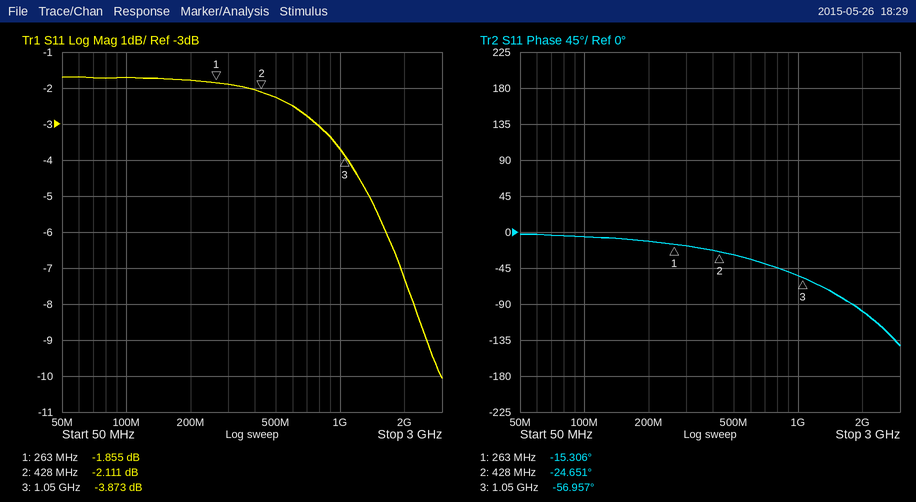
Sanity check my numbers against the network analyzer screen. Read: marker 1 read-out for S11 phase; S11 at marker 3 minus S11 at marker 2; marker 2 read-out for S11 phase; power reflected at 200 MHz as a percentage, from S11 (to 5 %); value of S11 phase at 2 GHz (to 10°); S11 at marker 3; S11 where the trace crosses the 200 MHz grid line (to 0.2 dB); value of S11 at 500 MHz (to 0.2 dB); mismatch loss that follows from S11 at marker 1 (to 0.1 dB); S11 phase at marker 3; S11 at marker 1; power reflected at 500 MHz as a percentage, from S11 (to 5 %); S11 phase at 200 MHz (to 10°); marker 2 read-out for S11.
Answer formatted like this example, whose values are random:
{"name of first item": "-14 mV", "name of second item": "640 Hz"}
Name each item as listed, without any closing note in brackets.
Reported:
{"marker 1 read-out for S11 phase": "-15.306°", "S11 at marker 3 minus S11 at marker 2": "-1.762 dB", "marker 2 read-out for S11 phase": "-24.651°", "power reflected at 200 MHz as a percentage, from S11": "65 %", "value of S11 phase at 2 GHz": "-100°", "S11 at marker 3": "-3.873 dB", "S11 where the trace crosses the 200 MHz grid line": "-1.8 dB", "value of S11 at 500 MHz": "-2.2 dB", "mismatch loss that follows from S11 at marker 1": "4.6 dB", "S11 phase at marker 3": "-56.957°", "S11 at marker 1": "-1.855 dB", "power reflected at 500 MHz as a percentage, from S11": "60 %", "S11 phase at 200 MHz": "-10°", "marker 2 read-out for S11": "-2.111 dB"}
